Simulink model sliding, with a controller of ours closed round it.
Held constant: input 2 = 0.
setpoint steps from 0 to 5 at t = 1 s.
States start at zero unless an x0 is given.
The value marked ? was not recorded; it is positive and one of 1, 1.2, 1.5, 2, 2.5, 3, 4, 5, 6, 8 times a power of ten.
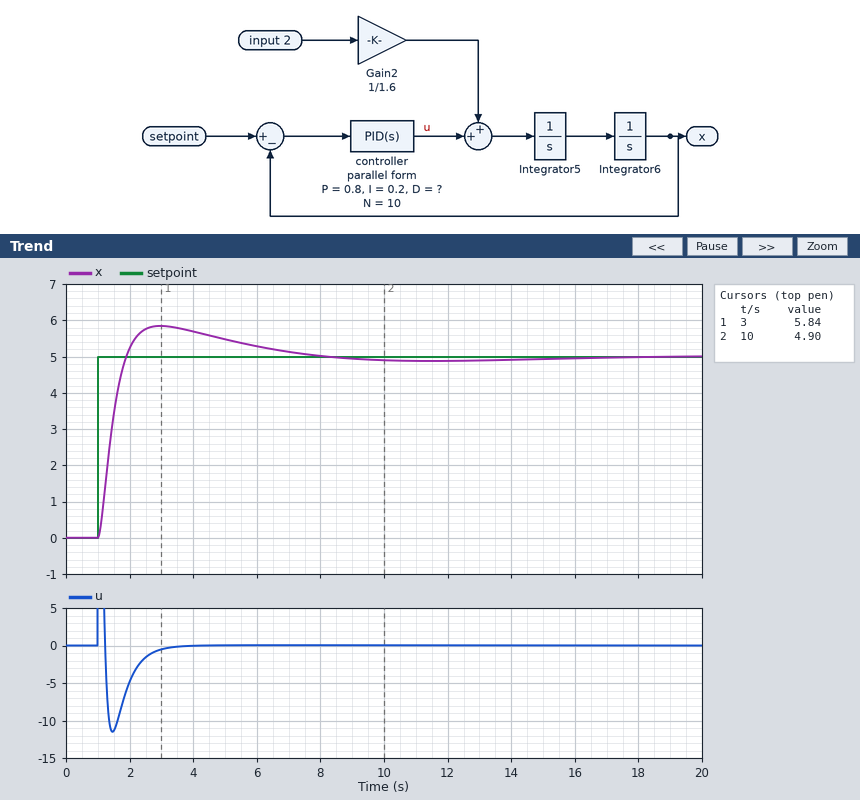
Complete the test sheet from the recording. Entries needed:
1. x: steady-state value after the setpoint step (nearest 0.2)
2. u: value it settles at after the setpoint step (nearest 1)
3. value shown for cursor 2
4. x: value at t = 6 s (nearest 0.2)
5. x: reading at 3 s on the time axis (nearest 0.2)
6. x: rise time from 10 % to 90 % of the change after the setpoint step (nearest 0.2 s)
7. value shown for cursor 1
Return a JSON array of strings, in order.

["5.0", "0", "4.90", "5.2", "5.8", "0.6 s", "5.84"]
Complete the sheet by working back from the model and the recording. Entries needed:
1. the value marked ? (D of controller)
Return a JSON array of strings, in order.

["2"]
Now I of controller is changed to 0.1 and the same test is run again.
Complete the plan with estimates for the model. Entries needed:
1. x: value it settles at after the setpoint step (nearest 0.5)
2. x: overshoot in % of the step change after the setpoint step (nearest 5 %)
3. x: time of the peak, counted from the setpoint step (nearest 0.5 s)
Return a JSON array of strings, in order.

["5.0", "15 %", "2.0 s"]
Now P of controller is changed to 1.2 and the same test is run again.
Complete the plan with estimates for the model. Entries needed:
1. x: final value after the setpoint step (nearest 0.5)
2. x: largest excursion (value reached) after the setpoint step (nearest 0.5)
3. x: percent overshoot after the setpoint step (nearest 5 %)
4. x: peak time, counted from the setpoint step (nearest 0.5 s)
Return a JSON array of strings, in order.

["5.0", "6.0", "20 %", "1.5 s"]
